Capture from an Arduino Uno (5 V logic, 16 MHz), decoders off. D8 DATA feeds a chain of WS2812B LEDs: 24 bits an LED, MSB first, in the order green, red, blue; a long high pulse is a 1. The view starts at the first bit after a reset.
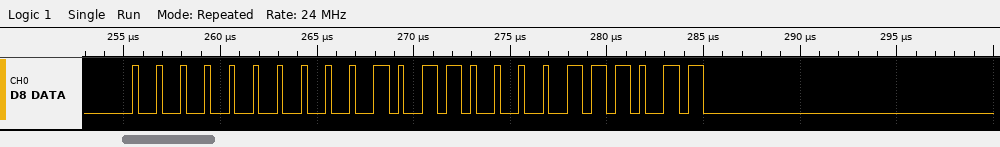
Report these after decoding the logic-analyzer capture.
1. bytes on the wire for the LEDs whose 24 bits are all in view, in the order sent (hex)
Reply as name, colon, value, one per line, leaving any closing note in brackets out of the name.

bytes on the wire for the LEDs whose 24 bits are all in view, in the order sent: 00 2C 3B
